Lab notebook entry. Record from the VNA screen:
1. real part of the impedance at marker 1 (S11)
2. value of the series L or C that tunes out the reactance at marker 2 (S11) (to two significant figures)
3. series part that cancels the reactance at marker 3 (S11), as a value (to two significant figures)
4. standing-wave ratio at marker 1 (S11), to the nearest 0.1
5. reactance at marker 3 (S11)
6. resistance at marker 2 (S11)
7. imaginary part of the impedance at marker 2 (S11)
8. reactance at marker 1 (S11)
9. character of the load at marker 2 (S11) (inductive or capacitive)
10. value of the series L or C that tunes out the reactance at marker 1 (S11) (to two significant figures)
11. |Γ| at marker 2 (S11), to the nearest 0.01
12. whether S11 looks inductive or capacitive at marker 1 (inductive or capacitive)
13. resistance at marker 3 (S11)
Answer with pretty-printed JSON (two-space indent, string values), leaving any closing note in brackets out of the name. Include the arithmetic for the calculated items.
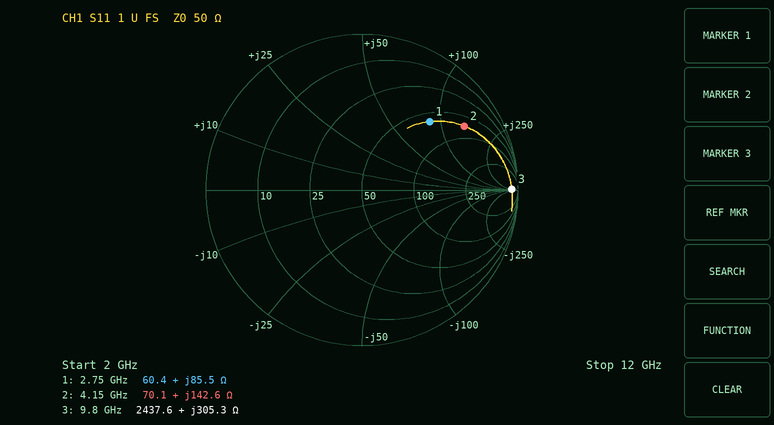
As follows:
{
  "real part of the impedance at marker 1": "60.4 Ω",
  "value of the series L or C that tunes out the reactance at marker 2 (S11)": "C = 1/(2π × 4.15 GHz × 142.6 Ω) ≈ 269 fF, so 270 fF to two significant figures",
  "series part that cancels the reactance at marker 3 (S11), as a value": "C = 1/(2π × 9.8 GHz × 305.3 Ω) ≈ 53 fF",
  "standing-wave ratio at marker 1 (S11), to the nearest 0.1": "4.2",
  "reactance at marker 3": "+305.3 Ω",
  "resistance at marker 2": "70.1 Ω",
  "imaginary part of the impedance at marker 2": "+142.6 Ω",
  "reactance at marker 1": "+85.5 Ω",
  "character of the load at marker 2 (S11)": "inductive",
  "value of the series L or C that tunes out the reactance at marker 1 (S11)": "C = 1/(2π × 2.75 GHz × 85.5 Ω) ≈ 677 fF, so 680 fF to two significant figures",
  "|Γ| at marker 2 (S11), to the nearest 0.01": "0.77",
  "whether S11 looks inductive or capacitive at marker 1": "inductive",
  "resistance at marker 3": "2437.6 Ω"
}
